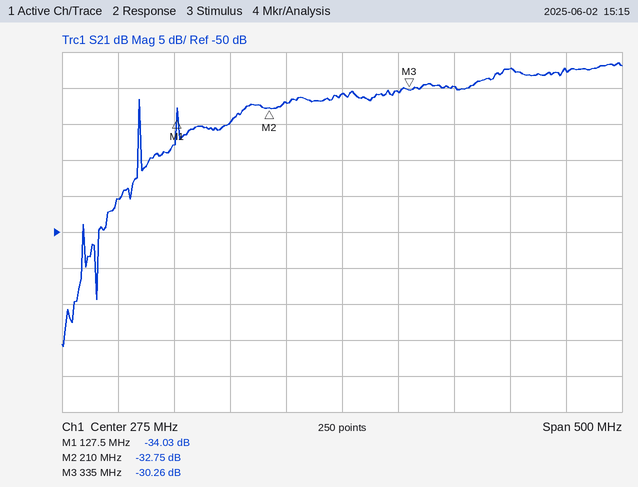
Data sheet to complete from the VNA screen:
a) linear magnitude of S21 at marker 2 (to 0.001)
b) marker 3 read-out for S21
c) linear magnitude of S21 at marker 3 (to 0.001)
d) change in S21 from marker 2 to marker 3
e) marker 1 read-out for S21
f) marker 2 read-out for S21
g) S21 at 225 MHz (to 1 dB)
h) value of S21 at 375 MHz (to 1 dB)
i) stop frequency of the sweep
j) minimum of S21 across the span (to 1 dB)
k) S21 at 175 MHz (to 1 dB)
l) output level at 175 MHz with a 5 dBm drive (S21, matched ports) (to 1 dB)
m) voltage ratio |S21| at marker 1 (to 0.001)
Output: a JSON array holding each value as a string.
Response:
["0.023", "-30.26 dB", "0.031", "2.49 dB", "-34.03 dB", "-32.75 dB", "-32 dB", "-30 dB", "525 MHz", "-66 dB", "-35 dB", "-30 dBm", "0.020"]
